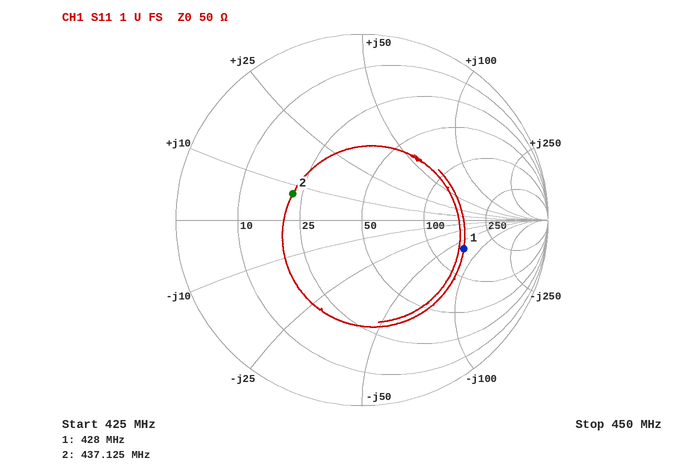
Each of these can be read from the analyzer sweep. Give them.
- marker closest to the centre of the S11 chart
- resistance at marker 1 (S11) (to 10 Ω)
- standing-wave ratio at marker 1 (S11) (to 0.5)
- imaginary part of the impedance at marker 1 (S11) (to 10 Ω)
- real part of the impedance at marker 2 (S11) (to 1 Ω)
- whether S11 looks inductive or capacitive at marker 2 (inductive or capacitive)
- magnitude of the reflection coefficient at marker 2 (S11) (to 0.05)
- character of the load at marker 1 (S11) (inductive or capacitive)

marker 2
150 Ω
3.5
-70 Ω
22 Ω
inductive
0.40
capacitive
